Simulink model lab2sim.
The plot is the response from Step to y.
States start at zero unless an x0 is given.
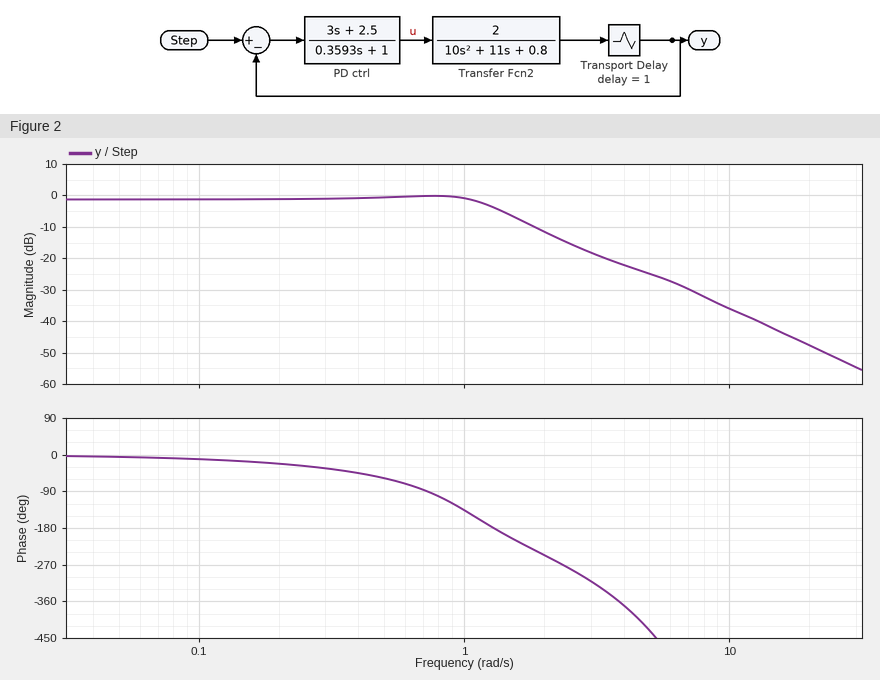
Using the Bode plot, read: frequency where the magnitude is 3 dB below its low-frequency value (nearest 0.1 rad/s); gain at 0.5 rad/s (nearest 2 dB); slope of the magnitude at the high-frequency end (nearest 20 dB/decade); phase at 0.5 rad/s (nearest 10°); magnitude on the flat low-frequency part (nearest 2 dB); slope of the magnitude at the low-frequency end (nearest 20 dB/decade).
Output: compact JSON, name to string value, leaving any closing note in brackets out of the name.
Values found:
{"frequency where the magnitude is 3 dB below its low-frequency value": "1.3 rad/s", "gain at 0.5 rad/s": "0 dB", "slope of the magnitude at the high-frequency end": "-40 dB/decade", "phase at 0.5 rad/s": "-60°", "magnitude on the flat low-frequency part": "-2 dB", "slope of the magnitude at the low-frequency end": "0 dB/decade"}
